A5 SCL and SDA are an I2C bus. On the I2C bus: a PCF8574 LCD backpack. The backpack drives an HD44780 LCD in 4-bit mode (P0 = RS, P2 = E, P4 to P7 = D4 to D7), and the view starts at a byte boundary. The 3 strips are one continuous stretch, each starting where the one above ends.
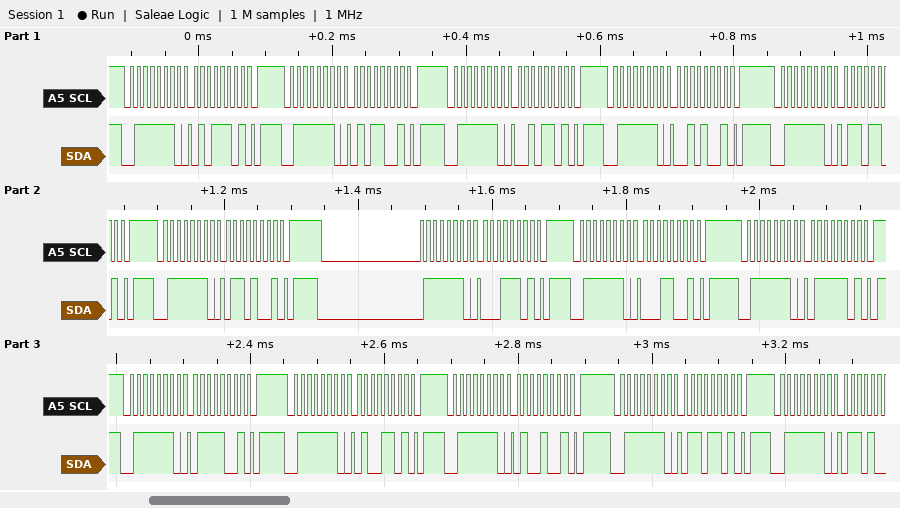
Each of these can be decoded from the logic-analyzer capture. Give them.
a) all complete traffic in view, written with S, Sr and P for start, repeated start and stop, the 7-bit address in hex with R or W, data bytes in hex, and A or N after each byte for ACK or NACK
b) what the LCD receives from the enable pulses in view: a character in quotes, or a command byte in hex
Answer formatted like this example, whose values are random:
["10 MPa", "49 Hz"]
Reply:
["S 3FW A 5D A P S 3FW A 59 A P S 3FW A 2D A P S 3FW A 29 A P S 3FW A 6D A P S 3FW A 69 A P S 3FW A 1D A P S 3FW A 19 A P S 3FW A 7D A P S 3FW A 79 A P S 3FW A 4D A P S 3FW A 49 A P S 3FW A 6D A P S 3FW A", "'R' 'a' 't'"]
